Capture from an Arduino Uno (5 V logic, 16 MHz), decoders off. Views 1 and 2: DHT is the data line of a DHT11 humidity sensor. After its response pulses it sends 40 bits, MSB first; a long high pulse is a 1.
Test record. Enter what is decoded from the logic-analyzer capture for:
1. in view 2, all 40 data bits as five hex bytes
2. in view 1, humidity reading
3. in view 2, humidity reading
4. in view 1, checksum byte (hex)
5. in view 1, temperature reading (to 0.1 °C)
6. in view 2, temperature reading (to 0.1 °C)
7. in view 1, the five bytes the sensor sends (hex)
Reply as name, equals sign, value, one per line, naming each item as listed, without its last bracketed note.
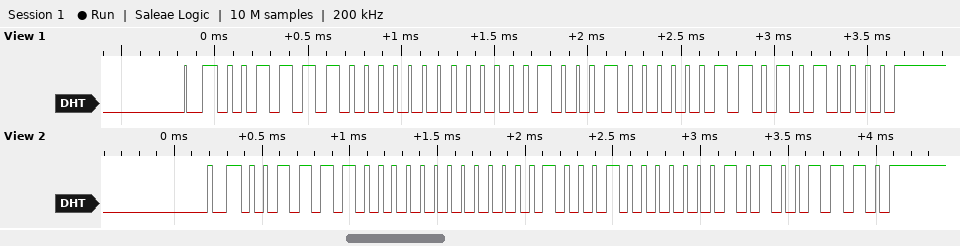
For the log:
in view 2, all 40 data bits as five hex bytes = 3C 00 11 01 4E
in view 1, humidity reading = 60 %
in view 2, humidity reading = 60 %
in view 1, checksum byte = 0x50
in view 1, temperature reading = 17.3 °C
in view 2, temperature reading = 17.1 °C
in view 1, the five bytes the sensor sends = 3C 00 11 03 50
